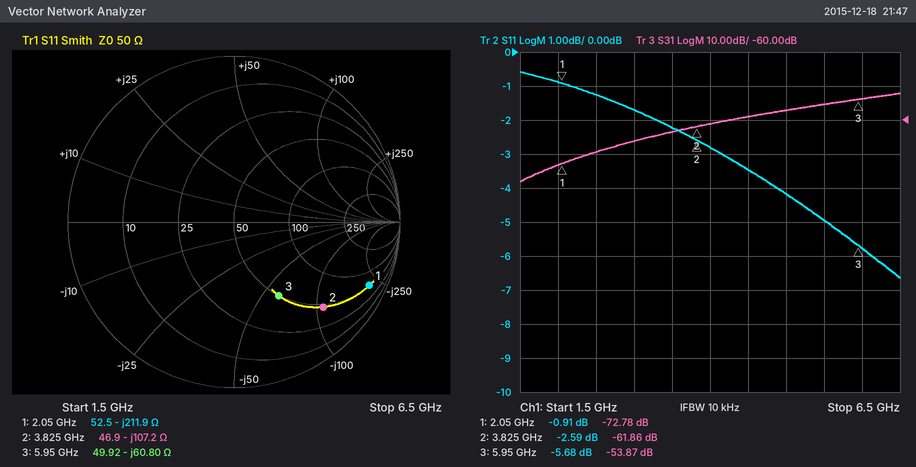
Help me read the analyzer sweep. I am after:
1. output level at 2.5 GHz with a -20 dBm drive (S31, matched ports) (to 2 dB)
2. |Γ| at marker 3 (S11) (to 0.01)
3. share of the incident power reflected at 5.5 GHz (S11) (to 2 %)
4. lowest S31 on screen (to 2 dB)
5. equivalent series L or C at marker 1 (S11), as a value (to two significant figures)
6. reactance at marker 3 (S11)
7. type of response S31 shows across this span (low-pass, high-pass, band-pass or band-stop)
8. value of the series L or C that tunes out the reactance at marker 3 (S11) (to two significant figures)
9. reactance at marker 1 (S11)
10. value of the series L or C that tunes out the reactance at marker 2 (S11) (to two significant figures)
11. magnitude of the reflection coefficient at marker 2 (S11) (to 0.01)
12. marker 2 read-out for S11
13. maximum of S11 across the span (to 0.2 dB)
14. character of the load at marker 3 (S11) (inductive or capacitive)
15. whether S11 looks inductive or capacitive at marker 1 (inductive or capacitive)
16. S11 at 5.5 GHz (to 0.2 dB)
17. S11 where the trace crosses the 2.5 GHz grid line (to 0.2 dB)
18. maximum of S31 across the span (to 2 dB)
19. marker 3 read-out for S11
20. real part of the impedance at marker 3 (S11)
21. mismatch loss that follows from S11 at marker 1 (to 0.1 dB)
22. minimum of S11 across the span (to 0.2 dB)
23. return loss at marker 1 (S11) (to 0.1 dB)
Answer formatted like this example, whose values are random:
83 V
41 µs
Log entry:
-90 dBm
0.52
32 %
-78 dB
370 fF
-60.80 Ω
high-pass
1.6 nH
-211.9 Ω
4.5 nH
0.74
-2.59 dB
-0.6 dB
capacitive
capacitive
-5.0 dB
-1.2 dB
-52 dB
-5.68 dB
49.92 Ω
7.2 dB
-6.6 dB
0.9 dB
